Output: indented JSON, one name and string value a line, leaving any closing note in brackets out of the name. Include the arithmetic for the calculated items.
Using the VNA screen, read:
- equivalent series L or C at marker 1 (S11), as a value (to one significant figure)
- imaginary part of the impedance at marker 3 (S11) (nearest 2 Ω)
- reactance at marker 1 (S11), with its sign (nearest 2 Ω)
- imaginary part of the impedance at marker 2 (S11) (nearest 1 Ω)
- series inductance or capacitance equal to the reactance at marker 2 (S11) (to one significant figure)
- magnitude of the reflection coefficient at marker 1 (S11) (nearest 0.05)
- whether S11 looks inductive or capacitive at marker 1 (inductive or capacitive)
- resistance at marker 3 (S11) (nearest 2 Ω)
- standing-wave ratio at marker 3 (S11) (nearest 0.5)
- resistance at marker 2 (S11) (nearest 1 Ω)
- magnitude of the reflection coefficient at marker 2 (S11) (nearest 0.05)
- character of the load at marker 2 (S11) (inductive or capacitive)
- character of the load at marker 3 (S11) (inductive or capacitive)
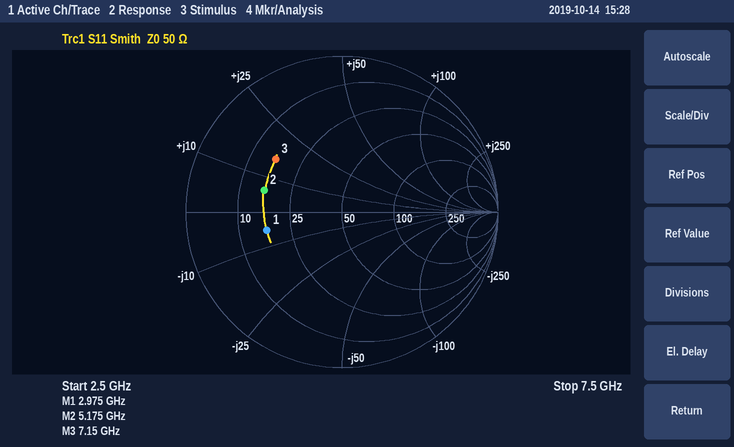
{
  "equivalent series L or C at marker 1 (S11), as a value": "C = 1/(2π × 2.975 GHz × 6 Ω) ≈ 8.92 pF, so 10 pF to one significant figure",
  "imaginary part of the impedance at marker 3 (S11)": "+16 Ω",
  "reactance at marker 1 (S11), with its sign": "-6 Ω",
  "imaginary part of the impedance at marker 2 (S11)": "+6 Ω",
  "series inductance or capacitance equal to the reactance at marker 2 (S11)": "L = 6 Ω/(2π × 5.175 GHz) ≈ 185 pH, so 200 pH to one significant figure",
  "magnitude of the reflection coefficient at marker 1 (S11)": "0.50",
  "whether S11 looks inductive or capacitive at marker 1": "capacitive",
  "resistance at marker 3 (S11)": "16 Ω",
  "standing-wave ratio at marker 3 (S11)": "3.5",
  "resistance at marker 2 (S11)": "16 Ω",
  "magnitude of the reflection coefficient at marker 2 (S11)": "0.50",
  "character of the load at marker 2 (S11)": "inductive",
  "character of the load at marker 3 (S11)": "inductive"
}
